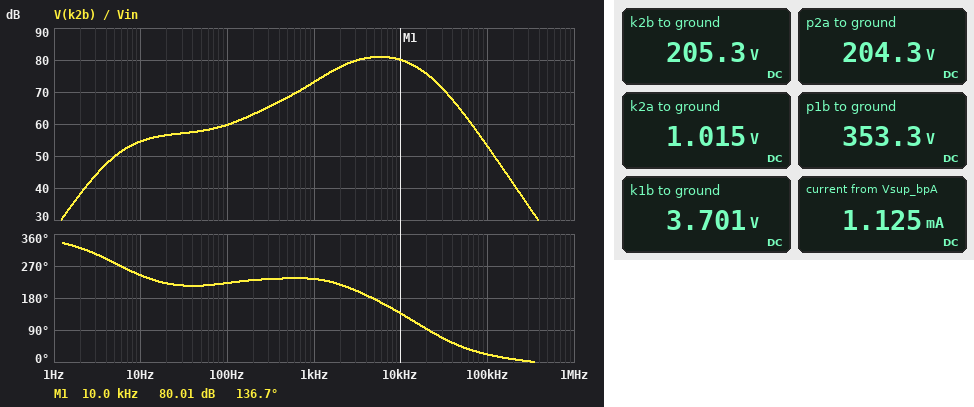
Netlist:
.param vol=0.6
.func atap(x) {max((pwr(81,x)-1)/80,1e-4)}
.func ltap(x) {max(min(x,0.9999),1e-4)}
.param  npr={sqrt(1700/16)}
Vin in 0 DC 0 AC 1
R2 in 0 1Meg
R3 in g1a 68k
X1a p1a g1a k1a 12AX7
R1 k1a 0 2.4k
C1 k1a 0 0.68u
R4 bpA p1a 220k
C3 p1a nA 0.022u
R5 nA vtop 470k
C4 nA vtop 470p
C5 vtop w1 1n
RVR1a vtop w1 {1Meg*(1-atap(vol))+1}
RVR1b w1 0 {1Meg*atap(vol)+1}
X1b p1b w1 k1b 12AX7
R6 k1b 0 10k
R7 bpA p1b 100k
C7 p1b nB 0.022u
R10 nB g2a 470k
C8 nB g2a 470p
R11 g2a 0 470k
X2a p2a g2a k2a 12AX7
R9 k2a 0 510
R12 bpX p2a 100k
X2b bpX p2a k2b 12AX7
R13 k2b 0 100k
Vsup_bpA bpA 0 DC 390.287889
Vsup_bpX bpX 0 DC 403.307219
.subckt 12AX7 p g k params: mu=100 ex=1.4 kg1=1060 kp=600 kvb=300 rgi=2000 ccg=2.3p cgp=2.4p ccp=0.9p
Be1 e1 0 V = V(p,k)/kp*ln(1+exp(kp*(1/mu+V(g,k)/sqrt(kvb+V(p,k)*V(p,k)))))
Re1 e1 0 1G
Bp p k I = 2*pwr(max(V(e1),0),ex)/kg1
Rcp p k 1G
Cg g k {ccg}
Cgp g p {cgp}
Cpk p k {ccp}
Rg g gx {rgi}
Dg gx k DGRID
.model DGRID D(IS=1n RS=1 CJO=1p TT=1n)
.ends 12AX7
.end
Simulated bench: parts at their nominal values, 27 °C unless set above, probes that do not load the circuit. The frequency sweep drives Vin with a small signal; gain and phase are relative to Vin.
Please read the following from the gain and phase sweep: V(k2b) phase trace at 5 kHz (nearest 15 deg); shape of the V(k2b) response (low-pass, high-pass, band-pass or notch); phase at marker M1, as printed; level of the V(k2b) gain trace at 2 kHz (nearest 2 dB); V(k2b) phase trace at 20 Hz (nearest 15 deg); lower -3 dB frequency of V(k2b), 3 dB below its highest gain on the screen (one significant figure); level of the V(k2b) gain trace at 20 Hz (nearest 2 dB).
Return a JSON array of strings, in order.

["180 deg", "band-pass", "136.7 deg", "78 dB", "225 deg", "2 kHz", "56 dB"]
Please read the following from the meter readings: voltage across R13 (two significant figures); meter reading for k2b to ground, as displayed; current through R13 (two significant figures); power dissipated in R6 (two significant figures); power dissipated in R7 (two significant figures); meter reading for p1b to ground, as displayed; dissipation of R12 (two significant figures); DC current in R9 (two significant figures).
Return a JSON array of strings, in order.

["210 V", "205.3 V", "2.1 mA", "1.4 mW", "14 mW", "353.3 V", "400 mW", "2.0 mA"]
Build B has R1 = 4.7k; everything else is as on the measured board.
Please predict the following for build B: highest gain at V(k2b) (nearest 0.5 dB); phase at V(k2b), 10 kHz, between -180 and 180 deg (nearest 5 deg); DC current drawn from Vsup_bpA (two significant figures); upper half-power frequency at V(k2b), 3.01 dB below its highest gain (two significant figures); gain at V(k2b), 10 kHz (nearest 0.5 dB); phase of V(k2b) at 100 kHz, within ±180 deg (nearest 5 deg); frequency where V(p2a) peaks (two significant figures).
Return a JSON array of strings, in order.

["79.5 dB", "140 deg", "910 µA", "16 kHz", "79.0 dB", "25 deg", "5.8 kHz"]
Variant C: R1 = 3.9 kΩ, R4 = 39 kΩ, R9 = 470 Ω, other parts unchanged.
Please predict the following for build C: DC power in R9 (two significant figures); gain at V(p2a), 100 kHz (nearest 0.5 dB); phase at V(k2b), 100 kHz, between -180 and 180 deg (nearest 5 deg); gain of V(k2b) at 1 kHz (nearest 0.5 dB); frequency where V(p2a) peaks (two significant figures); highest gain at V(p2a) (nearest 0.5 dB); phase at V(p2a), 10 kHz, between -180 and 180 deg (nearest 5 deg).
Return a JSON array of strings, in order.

["1.9 mW", "52.5 dB", "30 deg", "66.5 dB", "6.9 kHz", "75.5 dB", "150 deg"]
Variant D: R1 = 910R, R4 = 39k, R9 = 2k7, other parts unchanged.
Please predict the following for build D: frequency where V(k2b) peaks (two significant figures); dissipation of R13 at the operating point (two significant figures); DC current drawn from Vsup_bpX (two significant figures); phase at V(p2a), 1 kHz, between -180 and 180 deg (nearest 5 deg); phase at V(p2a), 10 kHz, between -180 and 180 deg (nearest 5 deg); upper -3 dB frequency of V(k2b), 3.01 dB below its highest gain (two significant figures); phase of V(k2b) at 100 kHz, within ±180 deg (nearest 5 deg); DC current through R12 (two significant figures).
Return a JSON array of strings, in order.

["7.8 kHz", "920 mW", "4.0 mA", "-110 deg", "160 deg", "23 kHz", "40 deg", "1.0 mA"]
